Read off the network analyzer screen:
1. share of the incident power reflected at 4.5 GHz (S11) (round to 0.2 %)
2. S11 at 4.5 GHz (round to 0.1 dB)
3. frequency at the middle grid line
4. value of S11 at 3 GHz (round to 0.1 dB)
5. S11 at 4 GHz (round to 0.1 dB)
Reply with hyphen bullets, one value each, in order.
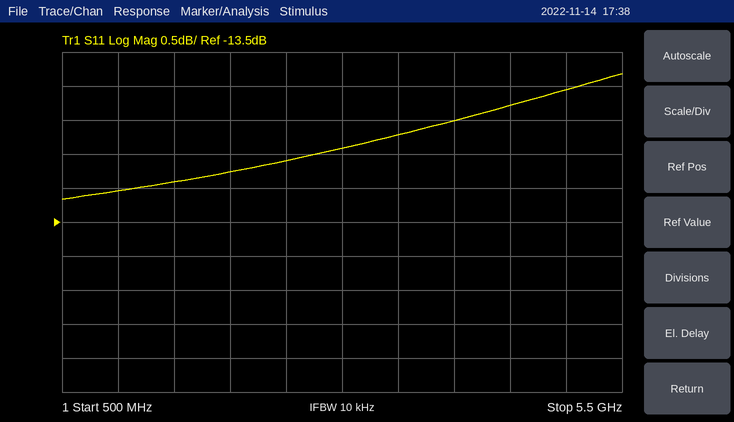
- 6.6 %
- -11.8 dB
- 3 GHz
- -12.4 dB
- -12.0 dB
